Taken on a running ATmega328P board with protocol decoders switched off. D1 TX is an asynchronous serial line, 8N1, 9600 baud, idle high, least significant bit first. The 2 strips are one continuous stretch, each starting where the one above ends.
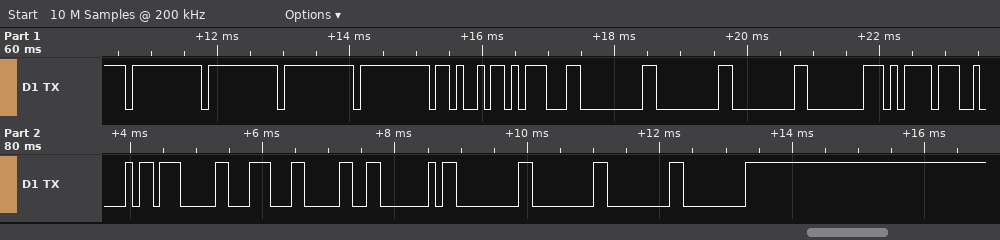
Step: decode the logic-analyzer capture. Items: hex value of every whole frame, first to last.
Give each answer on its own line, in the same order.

FF FF FF FF 4B 1D 00 00 00 80 BD 42 07 1C 30 40 00 00 00 00
